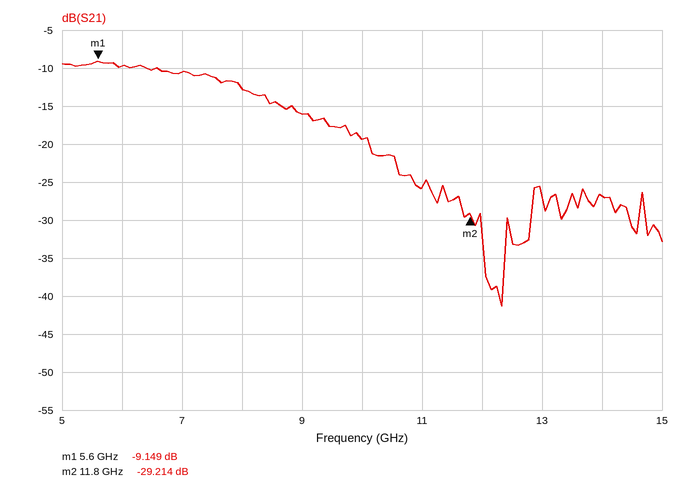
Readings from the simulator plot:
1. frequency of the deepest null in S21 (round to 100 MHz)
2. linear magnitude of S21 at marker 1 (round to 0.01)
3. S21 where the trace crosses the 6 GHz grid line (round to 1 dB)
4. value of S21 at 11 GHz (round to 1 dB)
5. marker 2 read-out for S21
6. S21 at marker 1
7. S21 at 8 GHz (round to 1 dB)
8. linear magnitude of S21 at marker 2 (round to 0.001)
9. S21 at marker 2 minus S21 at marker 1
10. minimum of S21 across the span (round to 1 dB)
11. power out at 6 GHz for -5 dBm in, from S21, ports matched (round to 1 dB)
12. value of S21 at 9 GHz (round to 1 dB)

12.3 GHz
0.35
-10 dB
-26 dB
-29.214 dB
-9.149 dB
-13 dB
0.035
-20.065 dB
-41 dB
-15 dBm
-16 dB
